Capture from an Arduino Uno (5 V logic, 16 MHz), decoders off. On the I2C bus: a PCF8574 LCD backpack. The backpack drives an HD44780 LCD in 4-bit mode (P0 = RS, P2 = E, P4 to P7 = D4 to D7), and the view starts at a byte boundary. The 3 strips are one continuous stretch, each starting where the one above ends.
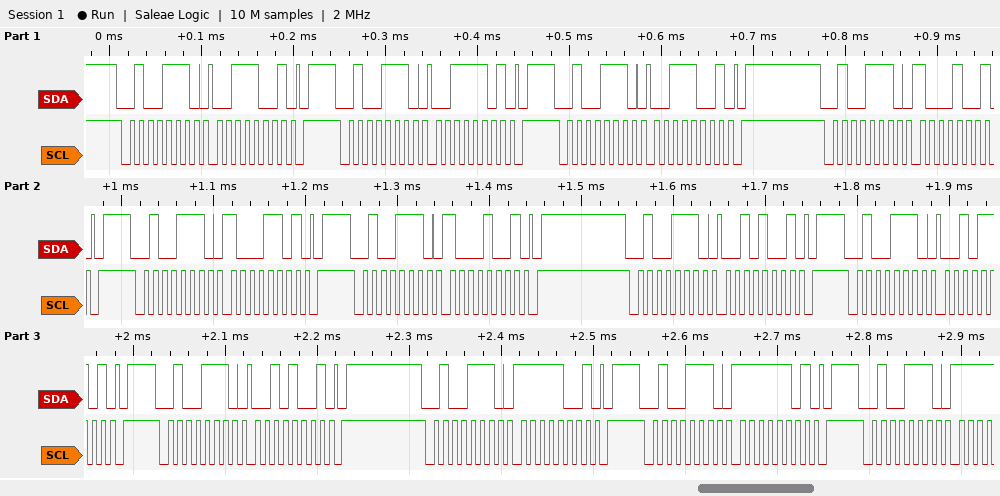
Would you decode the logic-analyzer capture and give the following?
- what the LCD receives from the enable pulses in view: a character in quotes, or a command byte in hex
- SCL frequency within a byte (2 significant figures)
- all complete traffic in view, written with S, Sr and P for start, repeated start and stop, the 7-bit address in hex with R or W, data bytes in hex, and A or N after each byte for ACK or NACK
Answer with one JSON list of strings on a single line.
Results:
["'8'", "100 kHz", "S 27W A 39 A P S 27W A 3D A P S 27W A 39 A P S 27W A 89 A P S 27W A 8D A P S 27W A 89 A P S 27W A 29 A P S 27W A 2D A P S 27W A 29 A P S 27W A F9 A P S 27W A FD A P S 27W A"]
